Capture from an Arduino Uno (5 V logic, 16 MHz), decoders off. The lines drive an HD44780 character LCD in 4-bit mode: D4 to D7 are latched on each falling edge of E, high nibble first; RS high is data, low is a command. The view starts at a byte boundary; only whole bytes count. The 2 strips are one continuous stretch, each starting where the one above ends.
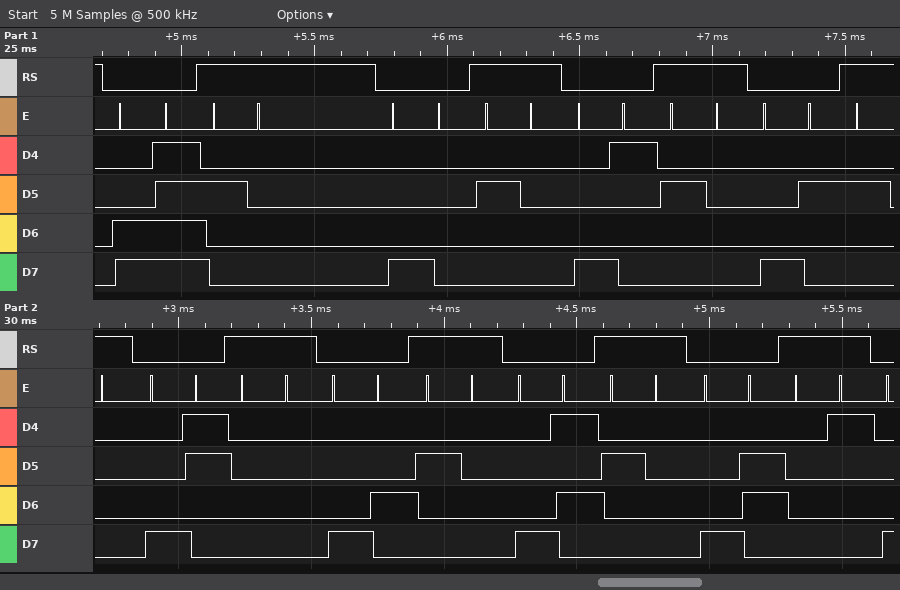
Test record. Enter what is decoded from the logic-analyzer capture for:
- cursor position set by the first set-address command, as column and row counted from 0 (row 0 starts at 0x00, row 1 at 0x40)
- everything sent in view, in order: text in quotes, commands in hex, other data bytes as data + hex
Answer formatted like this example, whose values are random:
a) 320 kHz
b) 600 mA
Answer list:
a) column 15, row 1
b) 0xCF " " 0x80 " " 0x81 " " 0x82 " " 0x83 data 00 0x84 " " 0x85 " " 0x86 data 01
